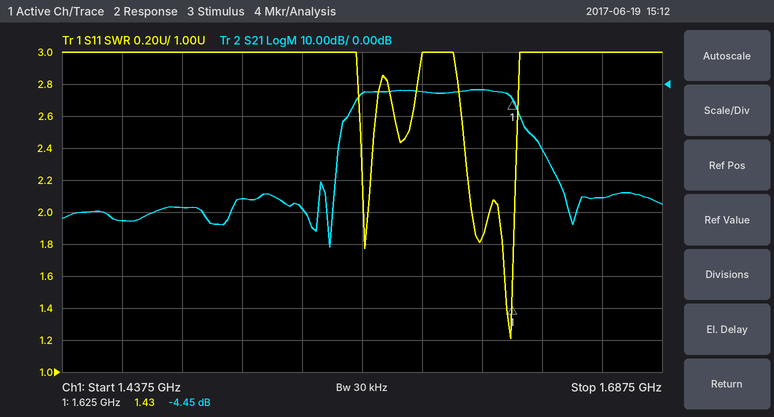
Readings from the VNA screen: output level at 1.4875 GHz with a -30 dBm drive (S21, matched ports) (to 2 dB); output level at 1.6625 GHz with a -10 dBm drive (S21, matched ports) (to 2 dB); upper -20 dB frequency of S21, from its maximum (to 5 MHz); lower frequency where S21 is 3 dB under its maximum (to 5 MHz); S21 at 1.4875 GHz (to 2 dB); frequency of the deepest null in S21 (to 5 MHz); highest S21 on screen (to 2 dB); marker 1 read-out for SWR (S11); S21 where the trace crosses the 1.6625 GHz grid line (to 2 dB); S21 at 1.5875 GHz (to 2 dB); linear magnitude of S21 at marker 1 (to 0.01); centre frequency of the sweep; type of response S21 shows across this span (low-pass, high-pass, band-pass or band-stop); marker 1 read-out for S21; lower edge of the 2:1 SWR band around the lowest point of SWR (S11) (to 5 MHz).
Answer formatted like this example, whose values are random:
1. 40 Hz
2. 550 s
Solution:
1. -68 dBm
2. -46 dBm
3. 1.640 GHz
4. 1.560 GHz
5. -38 dB
6. 1.550 GHz
7. -2 dB
8. 1.43
9. -36 dB
10. -2 dB
11. 0.60
12. 1.5625 GHz
13. band-pass
14. -4.45 dB
15. 1.620 GHz
